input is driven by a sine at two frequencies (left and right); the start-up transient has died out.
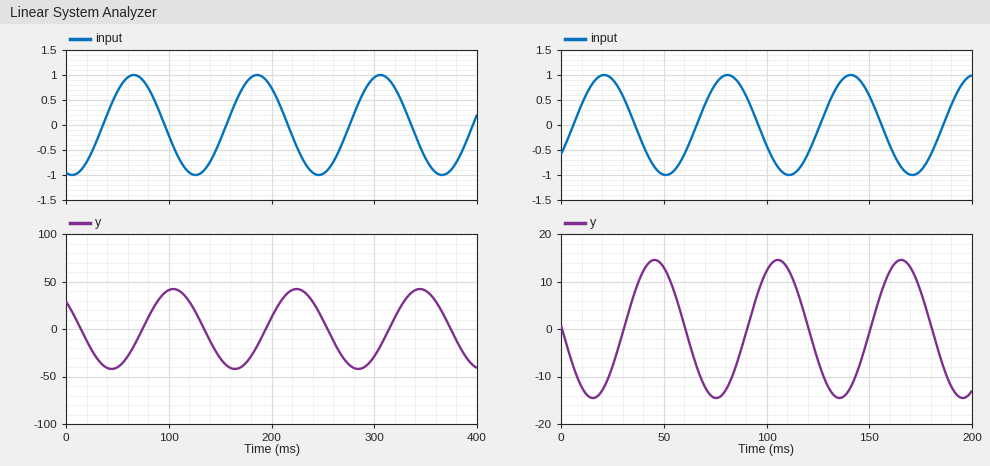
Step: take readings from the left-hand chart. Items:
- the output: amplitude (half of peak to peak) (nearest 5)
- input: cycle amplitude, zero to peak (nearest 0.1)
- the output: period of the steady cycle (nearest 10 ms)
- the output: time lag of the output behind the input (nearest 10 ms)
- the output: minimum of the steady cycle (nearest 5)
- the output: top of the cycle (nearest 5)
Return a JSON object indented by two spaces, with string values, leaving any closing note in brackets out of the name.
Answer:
{
  "the output: amplitude (half of peak to peak)": "40",
  "input: cycle amplitude, zero to peak": "1.0",
  "the output: period of the steady cycle": "120 ms",
  "the output: time lag of the output behind the input": "40 ms",
  "the output: minimum of the steady cycle": "-40",
  "the output: top of the cycle": "40"
}
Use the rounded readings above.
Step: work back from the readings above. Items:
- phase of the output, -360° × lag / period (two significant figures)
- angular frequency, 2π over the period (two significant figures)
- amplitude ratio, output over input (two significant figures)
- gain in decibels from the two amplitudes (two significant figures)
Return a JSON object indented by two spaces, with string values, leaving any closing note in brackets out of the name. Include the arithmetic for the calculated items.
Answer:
{
  "phase of the output, -360° × lag / period": "-360 × 40 / 120 = -120°",
  "angular frequency, 2π over the period": "2π / 120 = 0.052 rad/ms",
  "amplitude ratio, output over input": "40 / 1 = 40",
  "gain in decibels from the two amplitudes": "20 log10(40 / 1) = 32 dB"
}
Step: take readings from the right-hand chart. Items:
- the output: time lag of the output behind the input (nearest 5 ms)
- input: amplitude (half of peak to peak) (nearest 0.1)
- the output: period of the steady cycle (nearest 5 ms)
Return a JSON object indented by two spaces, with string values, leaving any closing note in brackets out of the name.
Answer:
{
  "the output: time lag of the output behind the input": "25 ms",
  "input: amplitude (half of peak to peak)": "1.0",
  "the output: period of the steady cycle": "60 ms"
}
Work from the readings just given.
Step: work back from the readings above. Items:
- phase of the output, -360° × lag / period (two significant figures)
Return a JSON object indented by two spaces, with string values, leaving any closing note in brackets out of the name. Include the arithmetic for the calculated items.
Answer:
{
  "phase of the output, -360° × lag / period": "-360 × 25 / 60 = -150°"
}
